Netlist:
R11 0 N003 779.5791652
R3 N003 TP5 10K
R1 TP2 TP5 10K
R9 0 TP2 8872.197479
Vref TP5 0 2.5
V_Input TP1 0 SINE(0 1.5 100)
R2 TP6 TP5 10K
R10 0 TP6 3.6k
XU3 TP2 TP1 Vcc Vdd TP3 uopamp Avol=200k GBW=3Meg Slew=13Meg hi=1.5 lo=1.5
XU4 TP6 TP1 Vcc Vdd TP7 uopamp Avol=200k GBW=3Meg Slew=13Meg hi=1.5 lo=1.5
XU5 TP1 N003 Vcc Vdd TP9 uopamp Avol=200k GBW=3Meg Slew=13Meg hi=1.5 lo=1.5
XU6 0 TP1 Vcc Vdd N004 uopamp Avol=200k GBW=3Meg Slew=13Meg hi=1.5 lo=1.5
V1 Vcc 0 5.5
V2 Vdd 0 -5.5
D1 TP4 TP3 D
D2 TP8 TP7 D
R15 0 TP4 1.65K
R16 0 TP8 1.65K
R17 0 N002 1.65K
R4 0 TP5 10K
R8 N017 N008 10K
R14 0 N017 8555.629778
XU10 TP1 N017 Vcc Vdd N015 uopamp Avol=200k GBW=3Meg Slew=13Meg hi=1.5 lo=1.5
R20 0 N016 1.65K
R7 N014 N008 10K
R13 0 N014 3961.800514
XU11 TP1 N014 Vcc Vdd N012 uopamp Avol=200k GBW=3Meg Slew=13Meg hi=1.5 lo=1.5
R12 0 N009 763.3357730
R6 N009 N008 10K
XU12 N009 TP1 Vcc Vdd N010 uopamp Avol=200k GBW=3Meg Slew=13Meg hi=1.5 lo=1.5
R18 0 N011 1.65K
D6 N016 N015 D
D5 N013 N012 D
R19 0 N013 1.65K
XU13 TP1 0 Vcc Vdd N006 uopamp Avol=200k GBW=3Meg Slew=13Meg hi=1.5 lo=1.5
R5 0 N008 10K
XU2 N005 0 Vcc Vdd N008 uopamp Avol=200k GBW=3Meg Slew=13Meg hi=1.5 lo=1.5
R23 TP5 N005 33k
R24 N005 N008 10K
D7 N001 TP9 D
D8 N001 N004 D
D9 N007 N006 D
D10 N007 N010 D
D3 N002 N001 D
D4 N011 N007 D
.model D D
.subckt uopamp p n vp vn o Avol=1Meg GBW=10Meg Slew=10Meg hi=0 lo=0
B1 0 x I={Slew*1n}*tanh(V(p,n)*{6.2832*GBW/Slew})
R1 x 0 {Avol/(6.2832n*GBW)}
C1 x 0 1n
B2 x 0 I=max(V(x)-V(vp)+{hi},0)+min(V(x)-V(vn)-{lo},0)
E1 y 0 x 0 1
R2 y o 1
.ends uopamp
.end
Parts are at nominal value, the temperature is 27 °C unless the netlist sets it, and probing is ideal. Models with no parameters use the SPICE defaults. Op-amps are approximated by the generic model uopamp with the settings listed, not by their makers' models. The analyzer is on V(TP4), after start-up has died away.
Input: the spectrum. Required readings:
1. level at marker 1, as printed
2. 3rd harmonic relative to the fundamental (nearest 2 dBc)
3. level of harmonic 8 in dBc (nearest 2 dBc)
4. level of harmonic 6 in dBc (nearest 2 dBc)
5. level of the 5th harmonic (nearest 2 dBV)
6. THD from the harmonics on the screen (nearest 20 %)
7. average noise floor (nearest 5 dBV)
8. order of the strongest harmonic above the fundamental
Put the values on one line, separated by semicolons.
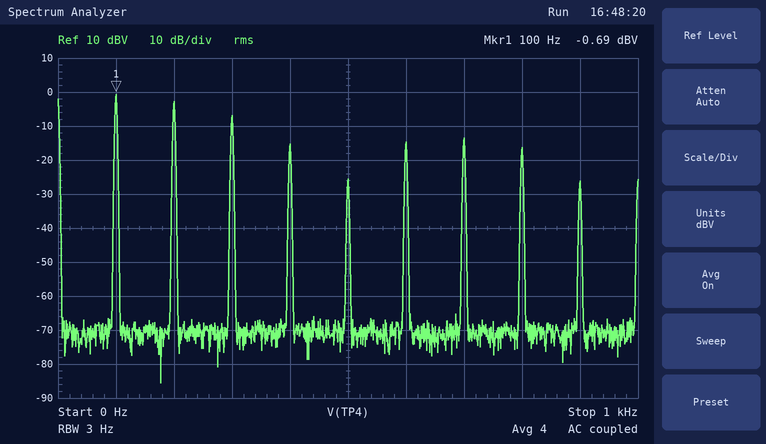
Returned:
-0.69 dBV; -6 dBc; -16 dBc; -14 dBc; -26 dBV; 100 %; -70 dBV; 2
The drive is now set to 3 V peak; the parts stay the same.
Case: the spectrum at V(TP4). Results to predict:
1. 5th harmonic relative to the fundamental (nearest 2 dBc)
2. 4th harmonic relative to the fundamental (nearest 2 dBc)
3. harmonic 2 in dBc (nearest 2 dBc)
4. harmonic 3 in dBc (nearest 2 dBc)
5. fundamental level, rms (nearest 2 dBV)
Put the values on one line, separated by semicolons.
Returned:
-20 dBc; -12 dBc; -8 dBc; -18 dBc; 2 dBV
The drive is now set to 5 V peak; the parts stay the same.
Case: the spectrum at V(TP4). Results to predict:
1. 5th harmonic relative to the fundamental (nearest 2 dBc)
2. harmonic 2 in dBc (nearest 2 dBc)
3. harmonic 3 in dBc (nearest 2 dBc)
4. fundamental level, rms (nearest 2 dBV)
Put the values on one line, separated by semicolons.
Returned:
-22 dBc; -12 dBc; -12 dBc; 4 dBV
